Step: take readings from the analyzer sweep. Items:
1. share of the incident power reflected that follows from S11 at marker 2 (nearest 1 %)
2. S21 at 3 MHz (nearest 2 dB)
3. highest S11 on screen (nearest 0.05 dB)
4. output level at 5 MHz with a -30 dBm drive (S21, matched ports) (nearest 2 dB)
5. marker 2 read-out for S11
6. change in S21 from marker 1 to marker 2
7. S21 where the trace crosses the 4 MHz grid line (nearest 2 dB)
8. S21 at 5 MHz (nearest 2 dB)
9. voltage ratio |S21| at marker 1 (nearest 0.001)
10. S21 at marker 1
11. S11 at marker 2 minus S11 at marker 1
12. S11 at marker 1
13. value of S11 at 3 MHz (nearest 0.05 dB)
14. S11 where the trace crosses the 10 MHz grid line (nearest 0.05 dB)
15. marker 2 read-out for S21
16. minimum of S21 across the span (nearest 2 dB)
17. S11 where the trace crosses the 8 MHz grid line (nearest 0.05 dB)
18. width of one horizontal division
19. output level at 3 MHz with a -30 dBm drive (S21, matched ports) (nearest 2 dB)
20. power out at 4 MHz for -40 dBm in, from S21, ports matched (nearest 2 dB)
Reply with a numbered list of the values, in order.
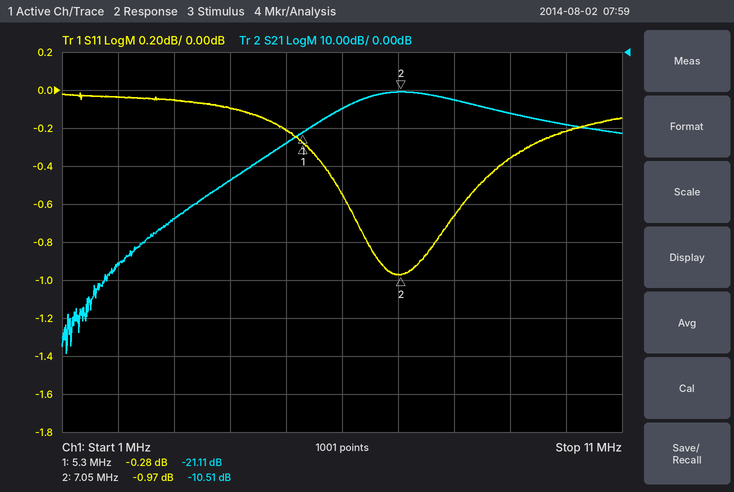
1. 80 %
2. -44 dB
3. 0.00 dB
4. -54 dBm
5. -0.97 dB
6. 10.60 dB
7. -34 dB
8. -24 dB
9. 0.088
10. -21.11 dB
11. -0.69 dB
12. -0.28 dB
13. -0.05 dB
14. -0.20 dB
15. -10.51 dB
16. -80 dB
17. -0.65 dB
18. 1 MHz
19. -74 dBm
20. -74 dBm
